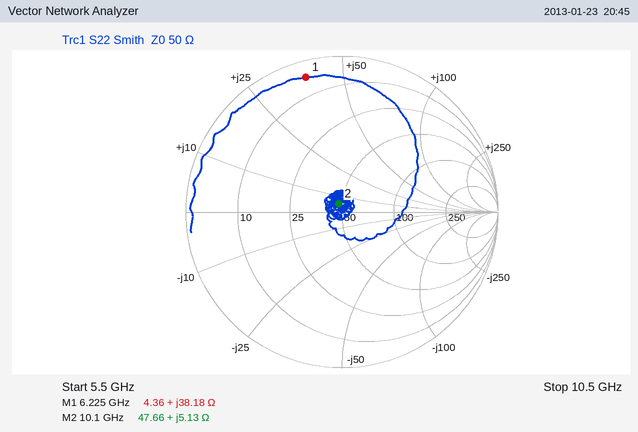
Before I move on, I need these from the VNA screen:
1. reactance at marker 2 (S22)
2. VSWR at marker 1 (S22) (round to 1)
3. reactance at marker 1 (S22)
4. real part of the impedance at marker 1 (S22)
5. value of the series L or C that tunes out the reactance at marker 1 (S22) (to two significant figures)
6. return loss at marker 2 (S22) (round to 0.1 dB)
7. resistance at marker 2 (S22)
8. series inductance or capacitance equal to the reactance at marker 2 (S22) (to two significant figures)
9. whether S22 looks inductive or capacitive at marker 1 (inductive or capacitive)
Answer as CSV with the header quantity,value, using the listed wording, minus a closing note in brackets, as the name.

quantity,value
reactance at marker 2,+5.13 Ω
VSWR at marker 1 (S22),18
reactance at marker 1,+38.18 Ω
real part of the impedance at marker 1,4.36 Ω
value of the series L or C that tunes out the reactance at marker 1 (S22),670 fF
return loss at marker 2 (S22),24.8 dB
resistance at marker 2,47.66 Ω
series inductance or capacitance equal to the reactance at marker 2 (S22),81 pH
whether S22 looks inductive or capacitive at marker 1,inductive
